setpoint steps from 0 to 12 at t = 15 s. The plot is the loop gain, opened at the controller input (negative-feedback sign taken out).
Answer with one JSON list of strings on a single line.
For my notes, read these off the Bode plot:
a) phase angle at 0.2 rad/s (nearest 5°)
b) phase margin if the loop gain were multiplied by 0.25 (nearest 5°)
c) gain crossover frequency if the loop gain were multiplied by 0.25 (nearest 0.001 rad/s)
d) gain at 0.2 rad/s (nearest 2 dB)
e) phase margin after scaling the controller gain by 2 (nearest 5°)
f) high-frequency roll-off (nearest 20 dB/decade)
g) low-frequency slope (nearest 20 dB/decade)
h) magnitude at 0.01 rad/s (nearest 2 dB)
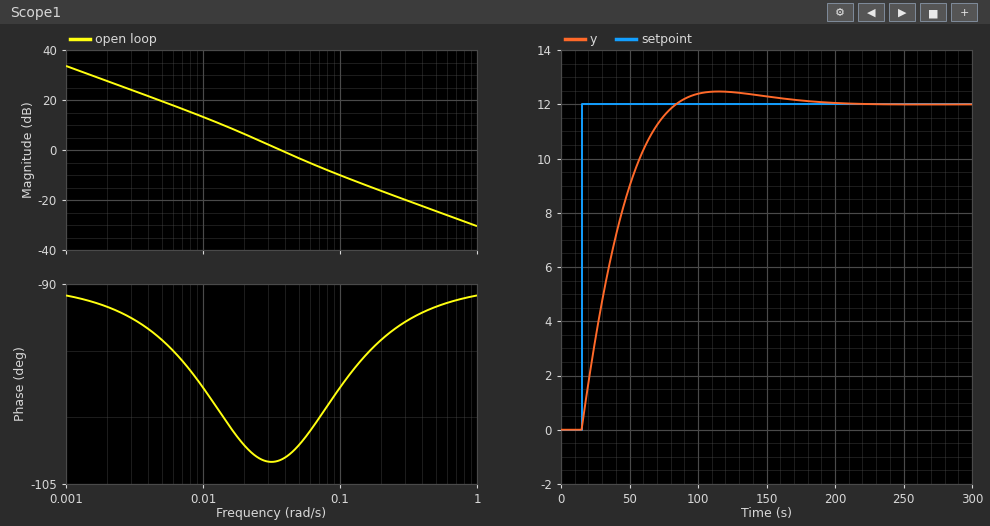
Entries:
["-95°", "80°", "0.011 rad/s", "-16 dB", "80°", "-20 dB/decade", "-20 dB/decade", "14 dB"]
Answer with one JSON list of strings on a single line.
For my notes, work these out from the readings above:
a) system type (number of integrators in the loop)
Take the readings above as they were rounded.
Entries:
["1"]
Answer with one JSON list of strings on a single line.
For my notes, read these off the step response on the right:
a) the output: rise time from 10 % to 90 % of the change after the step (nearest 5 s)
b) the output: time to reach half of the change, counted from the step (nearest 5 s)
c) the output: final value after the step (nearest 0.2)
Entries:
["45 s", "20 s", "12.0"]
